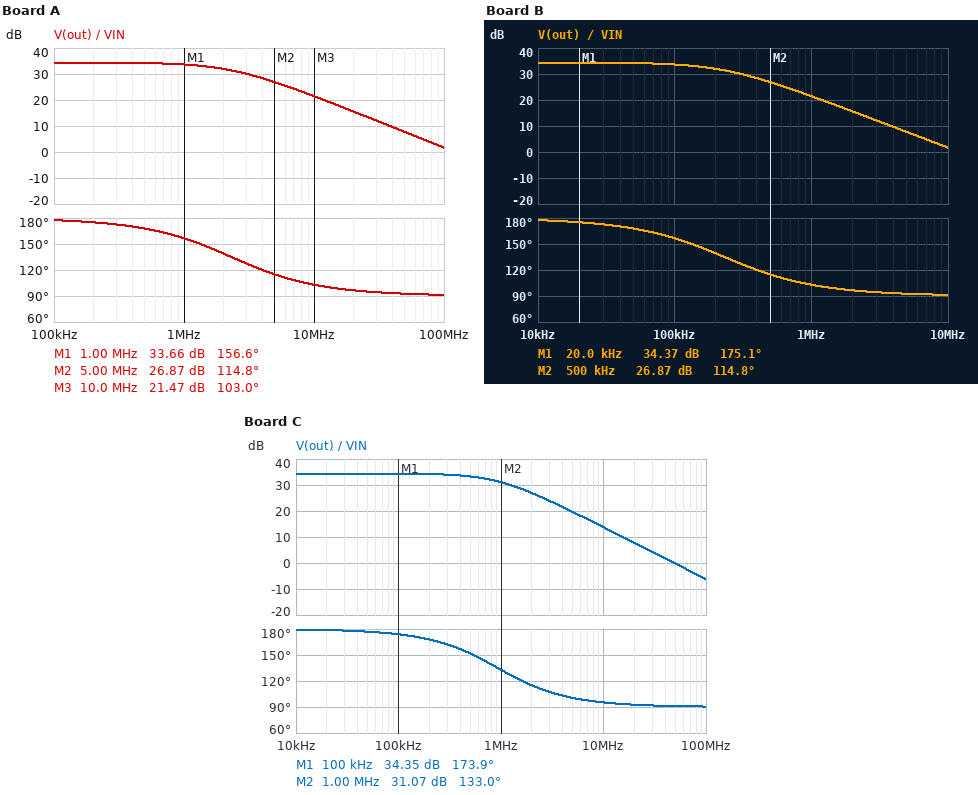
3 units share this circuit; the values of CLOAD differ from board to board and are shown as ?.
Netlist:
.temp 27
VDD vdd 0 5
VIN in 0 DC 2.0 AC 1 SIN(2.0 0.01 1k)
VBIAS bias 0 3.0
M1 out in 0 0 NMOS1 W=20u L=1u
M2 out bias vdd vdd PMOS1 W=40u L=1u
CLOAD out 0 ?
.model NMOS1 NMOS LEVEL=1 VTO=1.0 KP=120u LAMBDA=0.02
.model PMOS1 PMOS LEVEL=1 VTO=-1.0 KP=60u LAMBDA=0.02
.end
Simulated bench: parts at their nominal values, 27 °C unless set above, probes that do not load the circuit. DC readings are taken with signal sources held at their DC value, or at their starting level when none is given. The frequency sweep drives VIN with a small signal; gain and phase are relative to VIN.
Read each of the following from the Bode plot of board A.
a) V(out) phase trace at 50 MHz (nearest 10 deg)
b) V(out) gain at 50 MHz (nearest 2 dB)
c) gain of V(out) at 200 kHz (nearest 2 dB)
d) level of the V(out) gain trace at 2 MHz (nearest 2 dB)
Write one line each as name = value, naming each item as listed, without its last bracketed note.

V(out) phase trace at 50 MHz = 90 deg
V(out) gain at 50 MHz = 8 dB
gain of V(out) at 200 kHz = 34 dB
level of the V(out) gain trace at 2 MHz = 32 dB
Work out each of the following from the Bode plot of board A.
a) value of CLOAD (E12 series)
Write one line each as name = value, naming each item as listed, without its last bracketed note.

value of CLOAD = 3.3 pF
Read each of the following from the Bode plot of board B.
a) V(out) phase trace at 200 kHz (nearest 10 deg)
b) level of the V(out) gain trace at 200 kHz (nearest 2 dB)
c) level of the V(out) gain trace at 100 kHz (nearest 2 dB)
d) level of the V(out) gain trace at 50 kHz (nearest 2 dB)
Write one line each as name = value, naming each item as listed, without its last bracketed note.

V(out) phase trace at 200 kHz = 140 deg
level of the V(out) gain trace at 200 kHz = 32 dB
level of the V(out) gain trace at 100 kHz = 34 dB
level of the V(out) gain trace at 50 kHz = 34 dB
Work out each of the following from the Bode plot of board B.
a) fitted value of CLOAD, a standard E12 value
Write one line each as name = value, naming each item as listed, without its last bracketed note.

fitted value of CLOAD, a standard E12 value = 33 pF
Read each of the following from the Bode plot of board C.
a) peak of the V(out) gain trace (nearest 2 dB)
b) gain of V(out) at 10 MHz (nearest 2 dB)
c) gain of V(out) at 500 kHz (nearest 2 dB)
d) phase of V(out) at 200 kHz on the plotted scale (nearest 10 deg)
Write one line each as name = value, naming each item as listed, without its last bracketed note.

peak of the V(out) gain trace = 34 dB
gain of V(out) at 10 MHz = 14 dB
gain of V(out) at 500 kHz = 34 dB
phase of V(out) at 200 kHz on the plotted scale = 170 deg
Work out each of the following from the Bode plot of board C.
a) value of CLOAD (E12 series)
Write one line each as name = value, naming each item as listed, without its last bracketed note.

value of CLOAD = 8.2 pF
